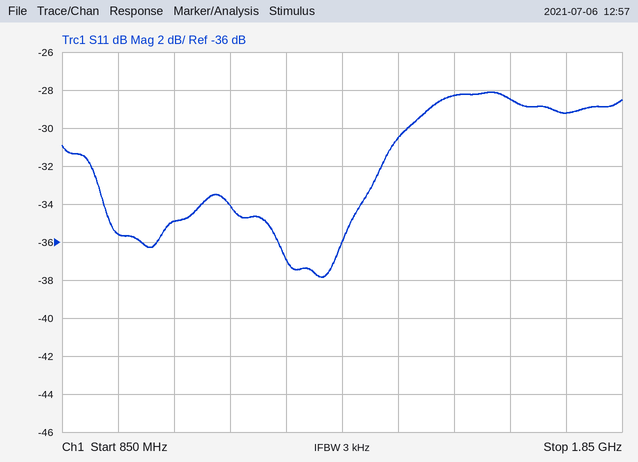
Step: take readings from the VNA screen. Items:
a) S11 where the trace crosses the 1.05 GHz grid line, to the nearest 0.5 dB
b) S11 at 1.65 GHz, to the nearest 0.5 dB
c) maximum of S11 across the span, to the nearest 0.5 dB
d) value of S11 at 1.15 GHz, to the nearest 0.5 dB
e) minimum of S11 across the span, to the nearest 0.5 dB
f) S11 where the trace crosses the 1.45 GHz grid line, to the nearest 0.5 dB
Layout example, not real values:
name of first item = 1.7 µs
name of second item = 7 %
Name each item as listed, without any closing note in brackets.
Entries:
S11 where the trace crosses the 1.05 GHz grid line, to the nearest 0.5 dB = -35.0 dB
S11 at 1.65 GHz, to the nearest 0.5 dB = -28.5 dB
maximum of S11 across the span, to the nearest 0.5 dB = -28.0 dB
value of S11 at 1.15 GHz, to the nearest 0.5 dB = -34.0 dB
minimum of S11 across the span, to the nearest 0.5 dB = -38.0 dB
S11 where the trace crosses the 1.45 GHz grid line, to the nearest 0.5 dB = -30.5 dB
